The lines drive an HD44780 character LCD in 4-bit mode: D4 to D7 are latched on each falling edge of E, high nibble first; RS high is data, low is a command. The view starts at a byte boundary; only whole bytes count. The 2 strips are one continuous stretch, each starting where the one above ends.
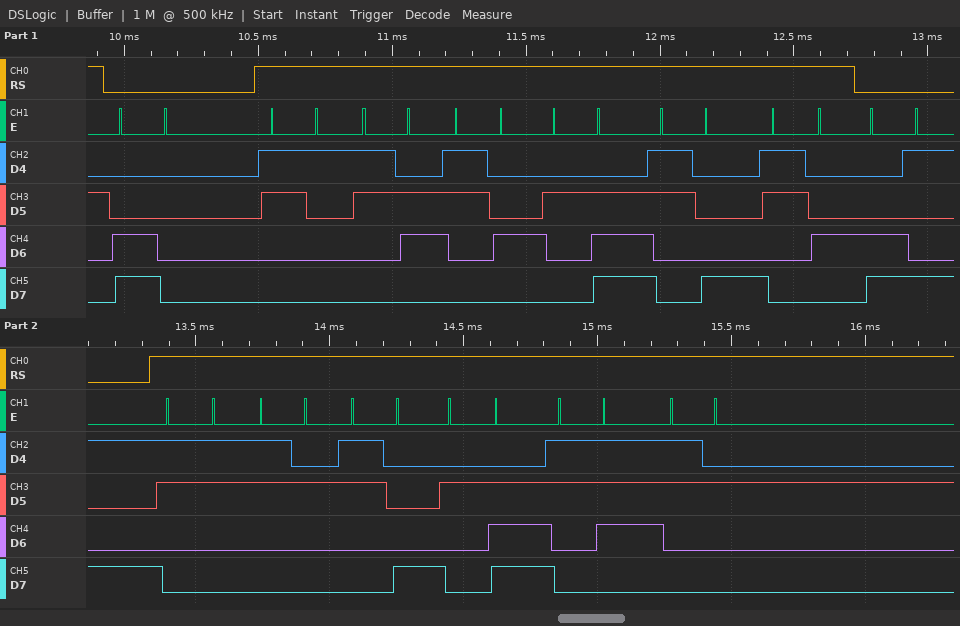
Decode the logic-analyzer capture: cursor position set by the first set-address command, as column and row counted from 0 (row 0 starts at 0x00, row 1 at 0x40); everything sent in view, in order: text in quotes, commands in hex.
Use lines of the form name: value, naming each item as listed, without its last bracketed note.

cursor position set by the first set-address command, as column and row counted from 0: column 0, row 1
everything sent in view, in order: text in quotes, commands in hex: 0xC0 "164.84" 0xC9 "328.72"
